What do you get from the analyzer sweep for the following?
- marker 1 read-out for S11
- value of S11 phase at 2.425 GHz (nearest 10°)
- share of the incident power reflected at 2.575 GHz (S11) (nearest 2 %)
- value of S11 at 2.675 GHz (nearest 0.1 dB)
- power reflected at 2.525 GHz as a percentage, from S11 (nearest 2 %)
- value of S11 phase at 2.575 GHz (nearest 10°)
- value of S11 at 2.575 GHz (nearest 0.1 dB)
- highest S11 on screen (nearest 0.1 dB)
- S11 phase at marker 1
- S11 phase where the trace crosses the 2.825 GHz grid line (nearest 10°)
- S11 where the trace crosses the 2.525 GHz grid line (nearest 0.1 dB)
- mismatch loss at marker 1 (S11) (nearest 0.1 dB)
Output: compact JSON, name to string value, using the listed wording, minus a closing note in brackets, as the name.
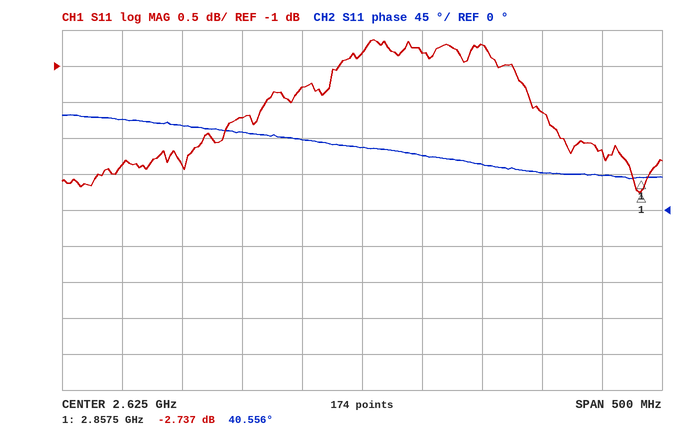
{"marker 1 read-out for S11": "-2.737 dB", "value of S11 phase at 2.425 GHz": "110°", "share of the incident power reflected at 2.575 GHz (S11)": "74 %", "value of S11 at 2.675 GHz": "-0.8 dB", "power reflected at 2.525 GHz as a percentage, from S11": "68 %", "value of S11 phase at 2.575 GHz": "90°", "value of S11 at 2.575 GHz": "-1.3 dB", "highest S11 on screen": "-0.6 dB", "S11 phase at marker 1": "40.556°", "S11 phase where the trace crosses the 2.825 GHz grid line": "40°", "S11 where the trace crosses the 2.525 GHz grid line": "-1.7 dB", "mismatch loss at marker 1 (S11)": "3.3 dB"}
